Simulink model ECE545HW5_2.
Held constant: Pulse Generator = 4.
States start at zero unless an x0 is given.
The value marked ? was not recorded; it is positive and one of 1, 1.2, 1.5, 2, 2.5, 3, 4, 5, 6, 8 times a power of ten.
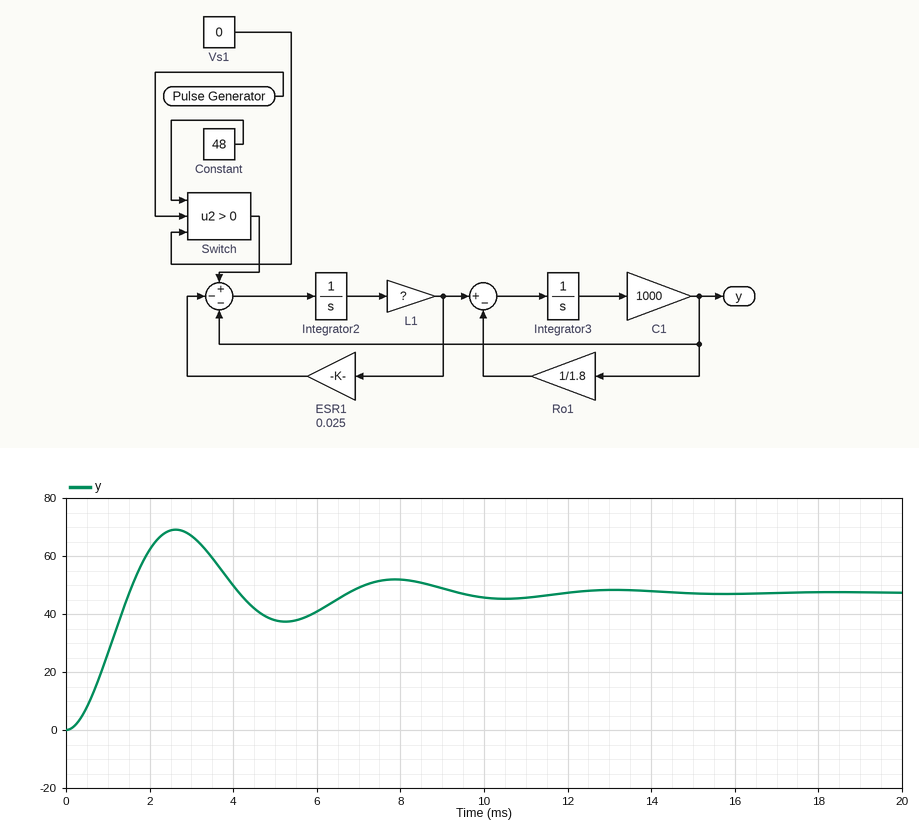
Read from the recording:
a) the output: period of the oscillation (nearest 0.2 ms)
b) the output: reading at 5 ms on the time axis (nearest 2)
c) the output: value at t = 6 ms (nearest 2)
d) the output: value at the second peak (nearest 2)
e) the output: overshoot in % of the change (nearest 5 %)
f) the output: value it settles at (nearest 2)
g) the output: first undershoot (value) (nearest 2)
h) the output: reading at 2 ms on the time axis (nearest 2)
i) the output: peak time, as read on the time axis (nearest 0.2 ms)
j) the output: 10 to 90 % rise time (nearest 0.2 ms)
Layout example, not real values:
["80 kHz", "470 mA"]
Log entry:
["5.2 ms", "38", "40", "52", "45 %", "48", "38", "62", "2.6 ms", "1.0 ms"]
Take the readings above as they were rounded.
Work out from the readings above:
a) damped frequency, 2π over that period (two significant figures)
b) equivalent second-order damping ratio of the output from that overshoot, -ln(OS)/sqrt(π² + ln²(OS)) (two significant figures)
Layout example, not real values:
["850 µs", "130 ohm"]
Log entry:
["1.2 rad/ms", "0.25"]
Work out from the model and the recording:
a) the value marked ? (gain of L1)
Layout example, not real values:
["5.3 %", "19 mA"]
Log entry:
["1500"]
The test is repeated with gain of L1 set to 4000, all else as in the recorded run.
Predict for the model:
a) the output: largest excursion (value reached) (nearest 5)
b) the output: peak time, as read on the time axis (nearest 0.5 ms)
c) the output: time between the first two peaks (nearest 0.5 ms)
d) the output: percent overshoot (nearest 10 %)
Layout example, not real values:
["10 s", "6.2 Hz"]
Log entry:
["75", "1.5 ms", "3.0 ms", "60 %"]
